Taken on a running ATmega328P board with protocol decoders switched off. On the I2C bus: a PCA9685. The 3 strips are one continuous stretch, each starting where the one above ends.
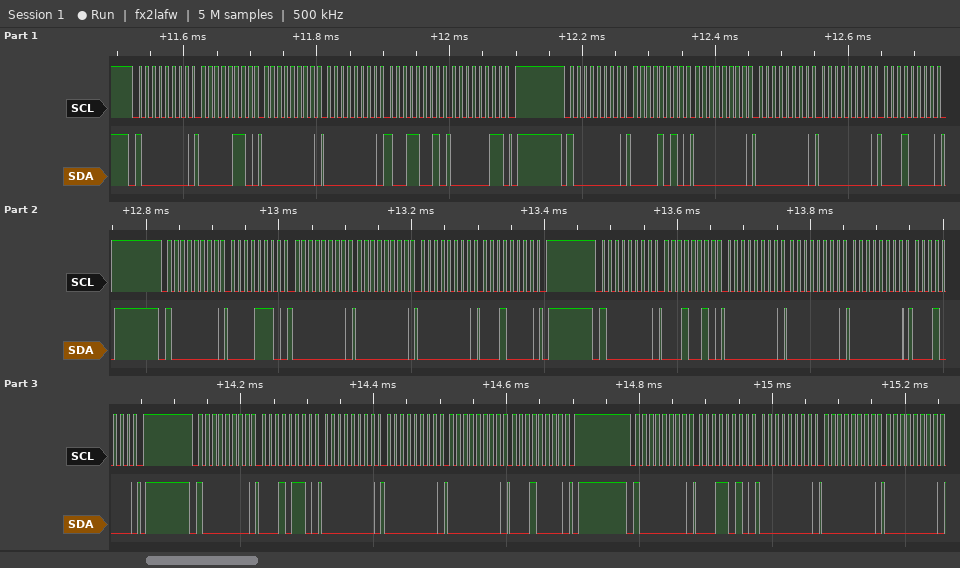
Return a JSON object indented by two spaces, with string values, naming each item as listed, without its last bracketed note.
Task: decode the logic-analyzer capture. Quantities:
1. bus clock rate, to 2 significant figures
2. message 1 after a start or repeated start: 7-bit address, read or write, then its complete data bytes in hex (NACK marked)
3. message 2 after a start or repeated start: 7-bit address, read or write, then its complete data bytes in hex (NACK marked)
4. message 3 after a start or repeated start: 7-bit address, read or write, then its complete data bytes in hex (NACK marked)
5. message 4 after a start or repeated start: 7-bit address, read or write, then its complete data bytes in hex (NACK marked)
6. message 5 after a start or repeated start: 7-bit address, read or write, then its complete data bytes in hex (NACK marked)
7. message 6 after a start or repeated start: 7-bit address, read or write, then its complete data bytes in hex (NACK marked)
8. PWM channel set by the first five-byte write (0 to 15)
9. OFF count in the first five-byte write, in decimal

{
  "bus clock rate, to 2 significant figures": "100 kHz",
  "message 1 after a start or repeated start: 7-bit address, read or write, then its complete data bytes in hex": "0x40 write: 06 00 00 99 03",
  "message 2 after a start or repeated start: 7-bit address, read or write, then its complete data bytes in hex": "0x40 write: 0A 00 00 00 10",
  "message 3 after a start or repeated start: 7-bit address, read or write, then its complete data bytes in hex": "0x40 write: 0E 00 00 00 10",
  "message 4 after a start or repeated start: 7-bit address, read or write, then its complete data bytes in hex": "0x40 write: 12 00 00 00 10",
  "message 5 after a start or repeated start: 7-bit address, read or write, then its complete data bytes in hex": "0x40 write: 16 00 00 00 10",
  "message 6 after a start or repeated start: 7-bit address, read or write, then its complete data bytes in hex": "0x40 write: 1A 00 00 00",
  "PWM channel set by the first five-byte write": "0",
  "OFF count in the first five-byte write, in decimal": "921"
}
